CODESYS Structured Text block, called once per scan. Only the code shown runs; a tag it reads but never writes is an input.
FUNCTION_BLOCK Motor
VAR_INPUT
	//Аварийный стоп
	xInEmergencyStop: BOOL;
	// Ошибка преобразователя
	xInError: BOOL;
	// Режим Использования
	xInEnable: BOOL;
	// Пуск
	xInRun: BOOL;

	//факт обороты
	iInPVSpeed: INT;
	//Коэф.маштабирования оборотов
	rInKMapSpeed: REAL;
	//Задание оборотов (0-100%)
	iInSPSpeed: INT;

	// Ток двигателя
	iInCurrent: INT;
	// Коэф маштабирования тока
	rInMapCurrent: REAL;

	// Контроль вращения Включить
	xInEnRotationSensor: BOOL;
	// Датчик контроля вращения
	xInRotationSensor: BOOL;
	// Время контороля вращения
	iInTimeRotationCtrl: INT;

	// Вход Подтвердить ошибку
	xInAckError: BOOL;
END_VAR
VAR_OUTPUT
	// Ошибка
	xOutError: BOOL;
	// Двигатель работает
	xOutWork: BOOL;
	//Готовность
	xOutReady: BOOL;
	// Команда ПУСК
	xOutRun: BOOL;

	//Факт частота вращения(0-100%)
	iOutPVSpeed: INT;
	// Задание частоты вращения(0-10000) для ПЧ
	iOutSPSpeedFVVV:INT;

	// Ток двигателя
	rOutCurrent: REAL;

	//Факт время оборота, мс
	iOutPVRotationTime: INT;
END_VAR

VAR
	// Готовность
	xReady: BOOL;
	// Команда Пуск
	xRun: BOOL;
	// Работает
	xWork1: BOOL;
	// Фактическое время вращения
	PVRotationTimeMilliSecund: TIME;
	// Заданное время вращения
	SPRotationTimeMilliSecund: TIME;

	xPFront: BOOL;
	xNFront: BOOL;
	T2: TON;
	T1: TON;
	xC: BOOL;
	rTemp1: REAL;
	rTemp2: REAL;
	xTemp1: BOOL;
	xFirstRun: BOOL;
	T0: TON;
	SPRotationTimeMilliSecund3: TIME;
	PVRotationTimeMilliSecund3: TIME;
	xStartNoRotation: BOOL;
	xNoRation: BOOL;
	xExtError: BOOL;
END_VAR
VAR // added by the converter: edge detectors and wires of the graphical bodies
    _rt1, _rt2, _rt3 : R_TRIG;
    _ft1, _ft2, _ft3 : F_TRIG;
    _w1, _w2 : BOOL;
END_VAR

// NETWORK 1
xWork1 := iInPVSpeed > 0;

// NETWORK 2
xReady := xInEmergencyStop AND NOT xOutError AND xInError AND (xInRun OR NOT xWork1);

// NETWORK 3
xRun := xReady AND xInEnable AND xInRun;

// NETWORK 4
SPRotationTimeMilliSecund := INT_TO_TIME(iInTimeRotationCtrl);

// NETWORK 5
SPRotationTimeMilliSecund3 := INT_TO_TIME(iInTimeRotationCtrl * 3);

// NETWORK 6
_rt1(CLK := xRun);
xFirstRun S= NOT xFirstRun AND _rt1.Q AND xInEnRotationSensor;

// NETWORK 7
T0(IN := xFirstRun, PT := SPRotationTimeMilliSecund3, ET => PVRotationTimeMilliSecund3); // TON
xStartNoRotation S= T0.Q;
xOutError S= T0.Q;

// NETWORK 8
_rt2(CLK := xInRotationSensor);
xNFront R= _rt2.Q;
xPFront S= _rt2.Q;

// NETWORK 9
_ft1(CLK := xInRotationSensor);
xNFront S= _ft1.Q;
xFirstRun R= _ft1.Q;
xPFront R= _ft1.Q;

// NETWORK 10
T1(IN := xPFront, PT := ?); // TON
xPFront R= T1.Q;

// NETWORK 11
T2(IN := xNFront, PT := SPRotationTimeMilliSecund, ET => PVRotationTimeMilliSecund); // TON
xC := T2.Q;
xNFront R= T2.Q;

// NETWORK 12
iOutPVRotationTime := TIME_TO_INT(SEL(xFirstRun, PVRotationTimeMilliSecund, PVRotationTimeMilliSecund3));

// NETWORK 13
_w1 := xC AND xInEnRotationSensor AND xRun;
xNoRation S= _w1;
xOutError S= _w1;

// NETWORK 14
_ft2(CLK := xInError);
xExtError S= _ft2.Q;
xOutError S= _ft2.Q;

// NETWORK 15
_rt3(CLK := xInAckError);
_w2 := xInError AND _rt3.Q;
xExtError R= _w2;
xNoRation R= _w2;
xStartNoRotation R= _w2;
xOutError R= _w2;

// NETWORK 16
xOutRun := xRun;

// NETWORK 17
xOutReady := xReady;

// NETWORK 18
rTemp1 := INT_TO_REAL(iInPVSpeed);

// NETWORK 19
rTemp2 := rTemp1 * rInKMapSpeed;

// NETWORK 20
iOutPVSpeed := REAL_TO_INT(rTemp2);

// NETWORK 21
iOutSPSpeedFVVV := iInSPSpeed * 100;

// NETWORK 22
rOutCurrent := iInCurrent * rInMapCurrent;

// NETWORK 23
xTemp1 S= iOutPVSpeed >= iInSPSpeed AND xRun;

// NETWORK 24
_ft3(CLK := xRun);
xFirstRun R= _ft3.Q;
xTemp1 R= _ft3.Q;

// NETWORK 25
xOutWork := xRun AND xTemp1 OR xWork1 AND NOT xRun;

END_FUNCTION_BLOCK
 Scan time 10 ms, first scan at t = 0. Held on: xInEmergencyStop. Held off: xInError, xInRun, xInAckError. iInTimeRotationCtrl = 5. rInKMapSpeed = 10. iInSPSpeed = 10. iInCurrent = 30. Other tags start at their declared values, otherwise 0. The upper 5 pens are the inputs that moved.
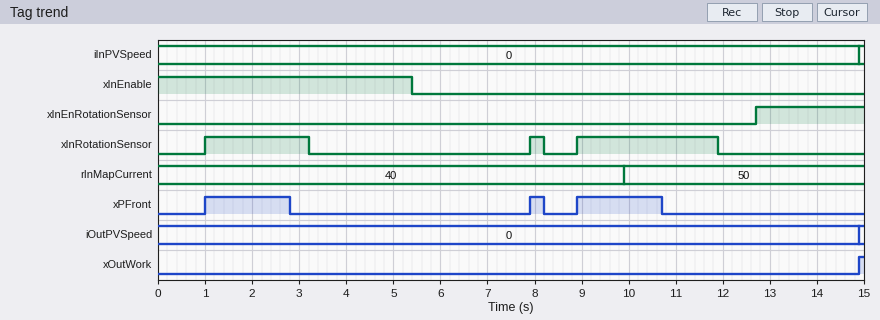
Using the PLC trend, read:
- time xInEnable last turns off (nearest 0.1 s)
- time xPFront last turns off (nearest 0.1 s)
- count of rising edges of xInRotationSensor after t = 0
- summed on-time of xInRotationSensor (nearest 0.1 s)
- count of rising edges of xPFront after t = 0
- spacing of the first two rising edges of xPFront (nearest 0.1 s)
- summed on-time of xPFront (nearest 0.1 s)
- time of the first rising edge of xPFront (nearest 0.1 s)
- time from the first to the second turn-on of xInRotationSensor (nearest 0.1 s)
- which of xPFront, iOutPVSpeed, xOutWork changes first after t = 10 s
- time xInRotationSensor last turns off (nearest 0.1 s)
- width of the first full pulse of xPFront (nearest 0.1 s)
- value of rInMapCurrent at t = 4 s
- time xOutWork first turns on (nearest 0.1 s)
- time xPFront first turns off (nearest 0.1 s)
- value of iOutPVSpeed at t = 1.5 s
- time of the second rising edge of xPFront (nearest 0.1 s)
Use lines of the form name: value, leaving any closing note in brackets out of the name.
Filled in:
time xInEnable last turns off: 5.4 s
time xPFront last turns off: 10.7 s
count of rising edges of xInRotationSensor after t = 0: 3
summed on-time of xInRotationSensor: 5.5 s
count of rising edges of xPFront after t = 0: 3
spacing of the first two rising edges of xPFront: 6.9 s
summed on-time of xPFront: 3.9 s
time of the first rising edge of xPFront: 1.0 s
time from the first to the second turn-on of xInRotationSensor: 6.9 s
which of xPFront, iOutPVSpeed, xOutWork changes first after t = 10 s: xPFront
time xInRotationSensor last turns off: 11.9 s
width of the first full pulse of xPFront: 1.8 s
value of rInMapCurrent at t = 4 s: 40
time xOutWork first turns on: 14.9 s
time xPFront first turns off: 2.8 s
value of iOutPVSpeed at t = 1.5 s: 0
time of the second rising edge of xPFront: 7.9 s
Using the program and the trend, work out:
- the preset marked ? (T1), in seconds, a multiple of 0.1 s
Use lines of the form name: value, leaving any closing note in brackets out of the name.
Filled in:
the preset marked ? (T1), in seconds, a multiple of 0.1 s: 1.8 s
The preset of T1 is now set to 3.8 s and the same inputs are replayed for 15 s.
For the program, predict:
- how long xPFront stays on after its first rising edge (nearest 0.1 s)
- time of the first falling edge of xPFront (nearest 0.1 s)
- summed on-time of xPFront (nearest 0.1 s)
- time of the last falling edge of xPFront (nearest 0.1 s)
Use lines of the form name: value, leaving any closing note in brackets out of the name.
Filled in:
how long xPFront stays on after its first rising edge: 2.2 s
time of the first falling edge of xPFront: 3.2 s
summed on-time of xPFront: 5.5 s
time of the last falling edge of xPFront: 11.9 s
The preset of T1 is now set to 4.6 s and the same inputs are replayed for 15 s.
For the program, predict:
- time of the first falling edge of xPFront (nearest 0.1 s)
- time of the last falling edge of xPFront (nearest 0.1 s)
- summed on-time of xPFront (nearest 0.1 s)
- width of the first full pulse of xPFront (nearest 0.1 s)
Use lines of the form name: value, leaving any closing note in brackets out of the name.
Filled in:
time of the first falling edge of xPFront: 3.2 s
time of the last falling edge of xPFront: 11.9 s
summed on-time of xPFront: 5.5 s
width of the first full pulse of xPFront: 2.2 s
